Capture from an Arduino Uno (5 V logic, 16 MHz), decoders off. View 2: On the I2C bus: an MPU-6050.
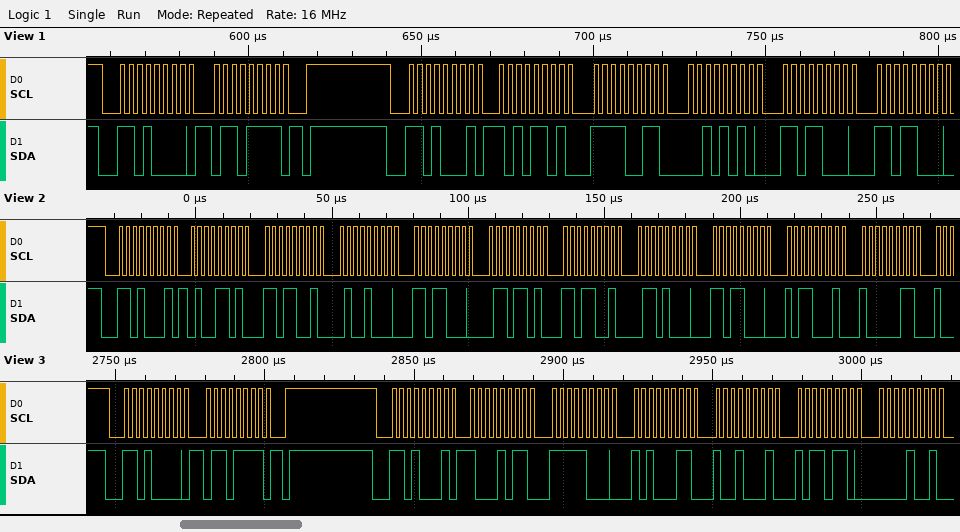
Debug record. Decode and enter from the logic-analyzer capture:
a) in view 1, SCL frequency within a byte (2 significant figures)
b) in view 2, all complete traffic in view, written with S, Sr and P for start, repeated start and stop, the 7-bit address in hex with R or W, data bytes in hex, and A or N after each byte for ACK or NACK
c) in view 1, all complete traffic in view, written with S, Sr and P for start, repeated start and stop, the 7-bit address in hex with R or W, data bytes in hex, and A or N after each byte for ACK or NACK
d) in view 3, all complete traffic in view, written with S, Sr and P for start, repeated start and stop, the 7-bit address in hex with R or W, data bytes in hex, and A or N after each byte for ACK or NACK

400 kHz
S 68R A 4D A D9 A 48 A D8 A 6D A D9 A 68 A D8 A B1 A 83 A
S 68W A 6F A P S 68R A AD A F3 A 2A A D8 A D8 A
S 68W A 6F A P S 68R A 8B A F8 A A3 A 91 A B6 A 09 A
